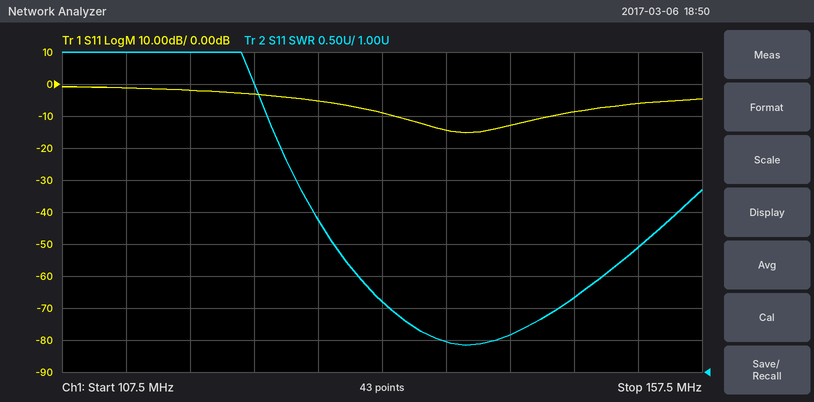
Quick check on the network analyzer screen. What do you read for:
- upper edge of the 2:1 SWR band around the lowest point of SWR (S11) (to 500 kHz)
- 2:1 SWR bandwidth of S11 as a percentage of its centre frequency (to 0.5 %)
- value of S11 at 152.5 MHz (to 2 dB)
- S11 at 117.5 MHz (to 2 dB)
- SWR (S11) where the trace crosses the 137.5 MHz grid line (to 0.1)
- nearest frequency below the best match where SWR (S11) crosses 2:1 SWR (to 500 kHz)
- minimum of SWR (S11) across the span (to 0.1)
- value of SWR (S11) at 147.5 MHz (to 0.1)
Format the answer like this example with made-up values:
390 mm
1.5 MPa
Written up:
146.5 MHz
9.5 %
-6 dB
-2 dB
1.5
133.0 MHz
1.4
2.2
